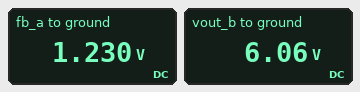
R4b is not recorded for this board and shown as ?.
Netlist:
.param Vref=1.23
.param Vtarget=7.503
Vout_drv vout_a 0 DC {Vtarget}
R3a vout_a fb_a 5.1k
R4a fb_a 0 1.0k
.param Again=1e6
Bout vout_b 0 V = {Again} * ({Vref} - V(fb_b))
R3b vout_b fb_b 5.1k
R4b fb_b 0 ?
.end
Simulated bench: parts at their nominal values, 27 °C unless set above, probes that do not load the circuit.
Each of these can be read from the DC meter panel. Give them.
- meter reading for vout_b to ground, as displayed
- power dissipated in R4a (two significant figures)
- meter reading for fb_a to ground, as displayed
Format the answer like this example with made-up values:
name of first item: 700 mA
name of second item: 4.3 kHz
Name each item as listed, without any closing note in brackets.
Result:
meter reading for vout_b to ground, as displayed: 6.06 V
power dissipated in R4a: 1.5 mW
meter reading for fb_a to ground, as displayed: 1.230 V
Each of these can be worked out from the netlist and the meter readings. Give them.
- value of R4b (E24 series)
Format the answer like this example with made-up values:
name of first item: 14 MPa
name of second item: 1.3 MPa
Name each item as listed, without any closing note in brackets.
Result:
value of R4b: 1.3 kΩ
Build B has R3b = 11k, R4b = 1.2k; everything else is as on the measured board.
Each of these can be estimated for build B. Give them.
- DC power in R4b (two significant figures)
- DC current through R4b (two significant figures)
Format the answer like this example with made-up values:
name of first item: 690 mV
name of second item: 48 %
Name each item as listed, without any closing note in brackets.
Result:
DC power in R4b: 1.3 mW
DC current through R4b: 1.0 mA
